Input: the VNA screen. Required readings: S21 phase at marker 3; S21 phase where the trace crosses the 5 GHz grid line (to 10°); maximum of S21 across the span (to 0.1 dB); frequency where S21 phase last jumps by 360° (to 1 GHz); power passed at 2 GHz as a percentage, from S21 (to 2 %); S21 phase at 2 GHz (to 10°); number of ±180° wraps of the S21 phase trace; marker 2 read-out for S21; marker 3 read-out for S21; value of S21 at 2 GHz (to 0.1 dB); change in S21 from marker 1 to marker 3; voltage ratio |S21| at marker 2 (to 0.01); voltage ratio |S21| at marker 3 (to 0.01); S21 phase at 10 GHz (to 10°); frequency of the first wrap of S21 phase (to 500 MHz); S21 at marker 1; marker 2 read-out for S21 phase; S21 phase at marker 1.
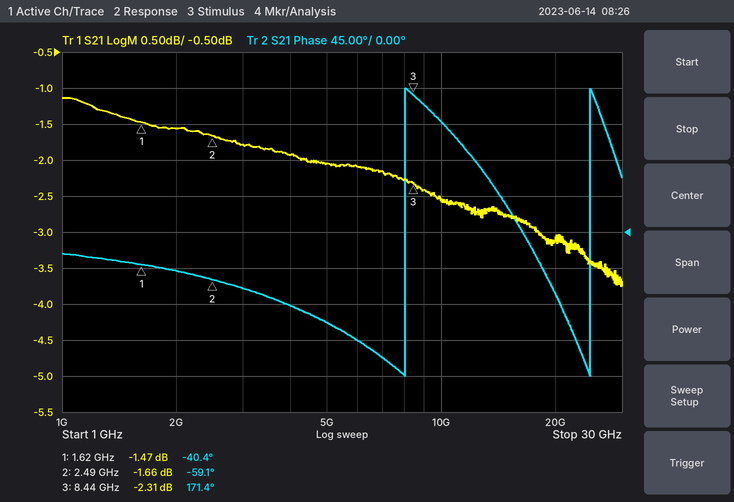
171.4°
-110°
-1.1 dB
25 GHz
70 %
-50°
2
-1.66 dB
-2.31 dB
-1.6 dB
-0.84 dB
0.83
0.77
140°
8.0 GHz
-1.47 dB
-59.1°
-40.4°
